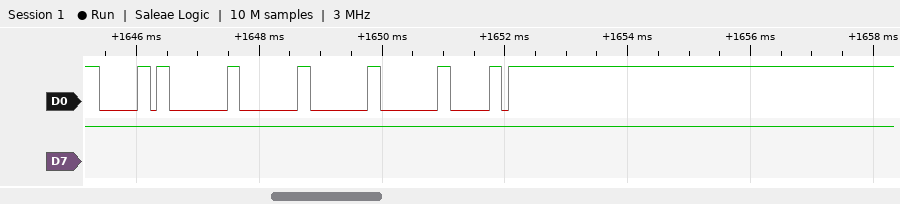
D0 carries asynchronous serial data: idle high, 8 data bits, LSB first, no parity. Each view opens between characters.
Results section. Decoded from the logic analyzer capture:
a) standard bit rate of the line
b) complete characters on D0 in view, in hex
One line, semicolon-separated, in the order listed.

9600 baud; 60, 00, 00, 00, 00, 60
